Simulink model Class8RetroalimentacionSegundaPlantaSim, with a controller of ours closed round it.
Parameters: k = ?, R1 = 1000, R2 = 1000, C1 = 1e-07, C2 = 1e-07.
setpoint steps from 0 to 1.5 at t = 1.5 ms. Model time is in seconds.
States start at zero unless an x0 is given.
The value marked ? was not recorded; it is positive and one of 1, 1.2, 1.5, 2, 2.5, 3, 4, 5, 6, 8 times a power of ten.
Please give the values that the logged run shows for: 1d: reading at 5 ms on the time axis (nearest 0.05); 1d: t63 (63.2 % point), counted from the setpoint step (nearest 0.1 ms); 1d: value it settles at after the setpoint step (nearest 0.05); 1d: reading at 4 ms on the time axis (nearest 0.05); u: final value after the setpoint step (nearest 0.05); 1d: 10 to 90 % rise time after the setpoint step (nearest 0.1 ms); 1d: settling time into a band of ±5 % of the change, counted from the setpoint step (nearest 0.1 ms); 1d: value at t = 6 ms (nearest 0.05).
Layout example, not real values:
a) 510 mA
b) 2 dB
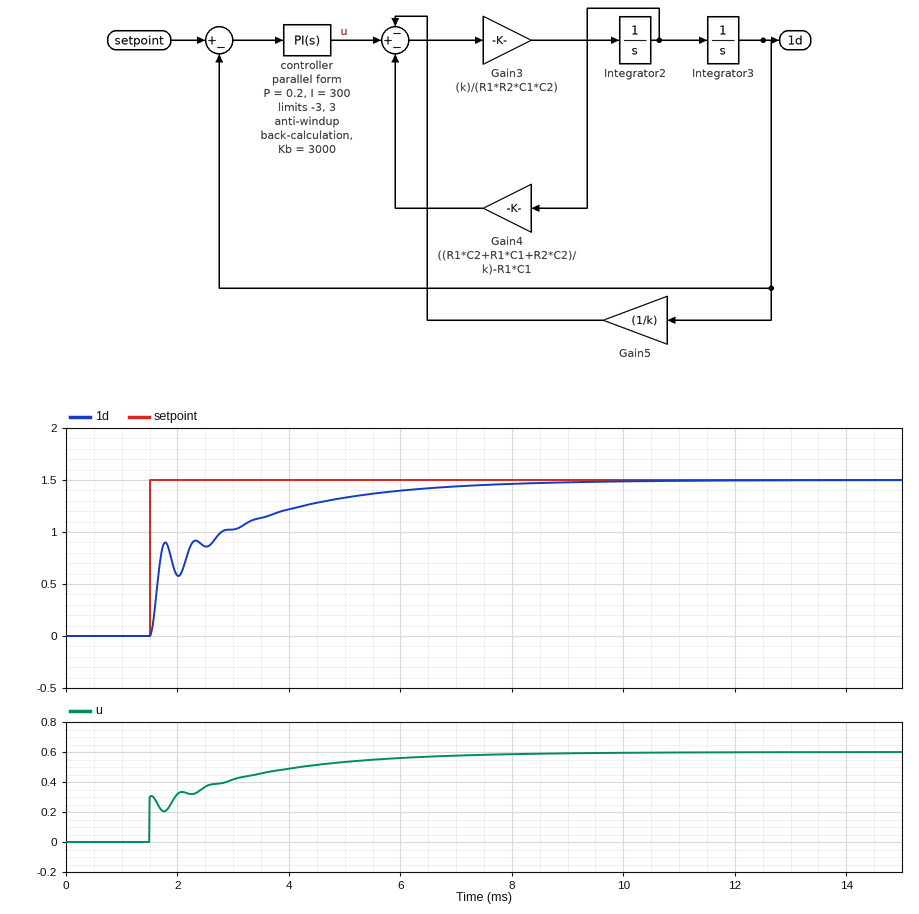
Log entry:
a) 1.35
b) 1.2 ms
c) 1.50
d) 1.20
e) 0.60
f) 3.7 ms
g) 5.1 ms
h) 1.40
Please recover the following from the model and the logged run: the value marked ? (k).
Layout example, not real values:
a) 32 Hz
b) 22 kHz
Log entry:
a) 2.5
